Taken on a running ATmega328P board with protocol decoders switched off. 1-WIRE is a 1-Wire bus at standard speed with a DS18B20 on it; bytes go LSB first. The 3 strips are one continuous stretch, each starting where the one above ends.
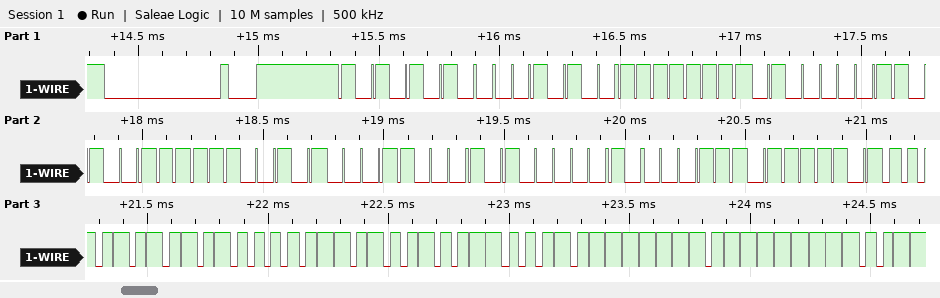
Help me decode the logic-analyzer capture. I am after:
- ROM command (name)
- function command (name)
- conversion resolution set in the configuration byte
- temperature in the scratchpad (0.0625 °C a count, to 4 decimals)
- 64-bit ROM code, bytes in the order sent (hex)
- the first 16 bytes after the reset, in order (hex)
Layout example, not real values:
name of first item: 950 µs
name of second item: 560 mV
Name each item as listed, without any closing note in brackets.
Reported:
ROM command: Match ROM
function command: Read Scratchpad
conversion resolution set in the configuration byte: 12 bits
temperature in the scratchpad: 85.0000 °C
64-bit ROM code, bytes in the order sent: 28 FF 82 E5 A7 18 05 E1
the first 16 bytes after the reset, in order: 55 28 FF 82 E5 A7 18 05 E1 BE 50 05 4B 46 7F FF
